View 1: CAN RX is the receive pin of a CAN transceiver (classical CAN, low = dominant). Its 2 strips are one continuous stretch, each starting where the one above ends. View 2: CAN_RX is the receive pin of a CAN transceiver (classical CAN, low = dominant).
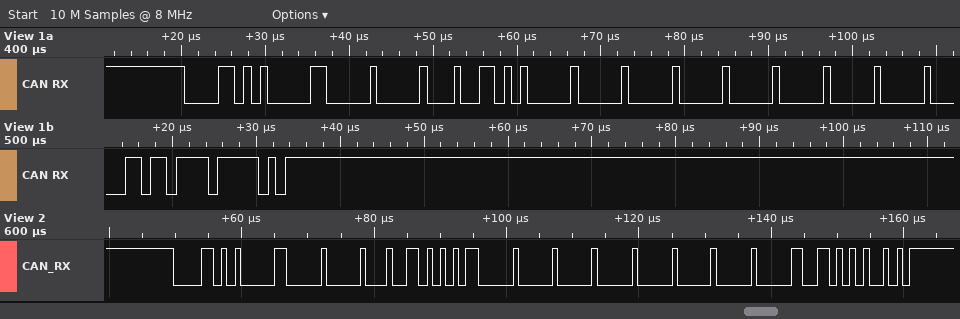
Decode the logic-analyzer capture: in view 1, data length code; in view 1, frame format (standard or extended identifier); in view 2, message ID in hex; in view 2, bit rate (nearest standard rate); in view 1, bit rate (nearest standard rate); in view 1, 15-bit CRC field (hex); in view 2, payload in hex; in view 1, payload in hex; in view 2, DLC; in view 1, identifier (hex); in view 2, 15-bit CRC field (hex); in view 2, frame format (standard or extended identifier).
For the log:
8
standard
0x0D4
1000 kbit/s
1000 kbit/s
0x5BDF
00 26 AB 00 00 00 00 00
00 26 A0 00 00 00 00 00
8
0x0D4
0x4D52
standard
